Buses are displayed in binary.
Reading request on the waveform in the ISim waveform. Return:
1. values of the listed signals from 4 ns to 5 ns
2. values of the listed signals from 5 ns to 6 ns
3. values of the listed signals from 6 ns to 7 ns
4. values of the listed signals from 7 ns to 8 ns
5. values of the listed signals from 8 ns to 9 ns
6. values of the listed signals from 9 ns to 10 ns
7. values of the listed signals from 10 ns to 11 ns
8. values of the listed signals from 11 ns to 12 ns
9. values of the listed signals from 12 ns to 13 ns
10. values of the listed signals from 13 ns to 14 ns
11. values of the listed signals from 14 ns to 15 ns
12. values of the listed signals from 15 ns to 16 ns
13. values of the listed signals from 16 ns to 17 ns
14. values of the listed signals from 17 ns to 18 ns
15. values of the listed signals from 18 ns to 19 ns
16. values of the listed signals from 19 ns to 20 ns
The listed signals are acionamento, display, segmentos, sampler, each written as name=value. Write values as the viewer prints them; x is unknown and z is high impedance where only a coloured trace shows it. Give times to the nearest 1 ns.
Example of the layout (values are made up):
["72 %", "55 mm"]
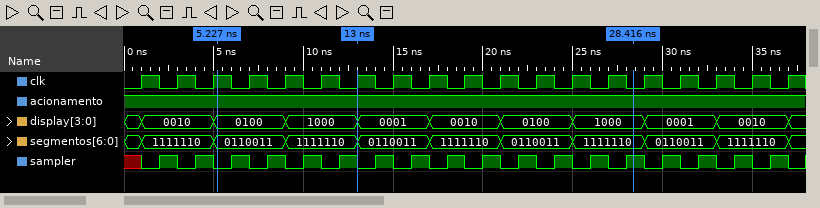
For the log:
["acionamento=1, display=0010, segmentos=1111110, sampler=1", "acionamento=1, display=0100, segmentos=0110011, sampler=0", "acionamento=1, display=0100, segmentos=0110011, sampler=1", "acionamento=1, display=0100, segmentos=0110011, sampler=0", "acionamento=1, display=0100, segmentos=0110011, sampler=1", "acionamento=1, display=1000, segmentos=1111110, sampler=0", "acionamento=1, display=1000, segmentos=1111110, sampler=1", "acionamento=1, display=1000, segmentos=1111110, sampler=0", "acionamento=1, display=1000, segmentos=1111110, sampler=1", "acionamento=1, display=0001, segmentos=0110011, sampler=0", "acionamento=1, display=0001, segmentos=0110011, sampler=1", "acionamento=1, display=0001, segmentos=0110011, sampler=0", "acionamento=1, display=0001, segmentos=0110011, sampler=1", "acionamento=1, display=0010, segmentos=1111110, sampler=0", "acionamento=1, display=0010, segmentos=1111110, sampler=1", "acionamento=1, display=0010, segmentos=1111110, sampler=0"]
